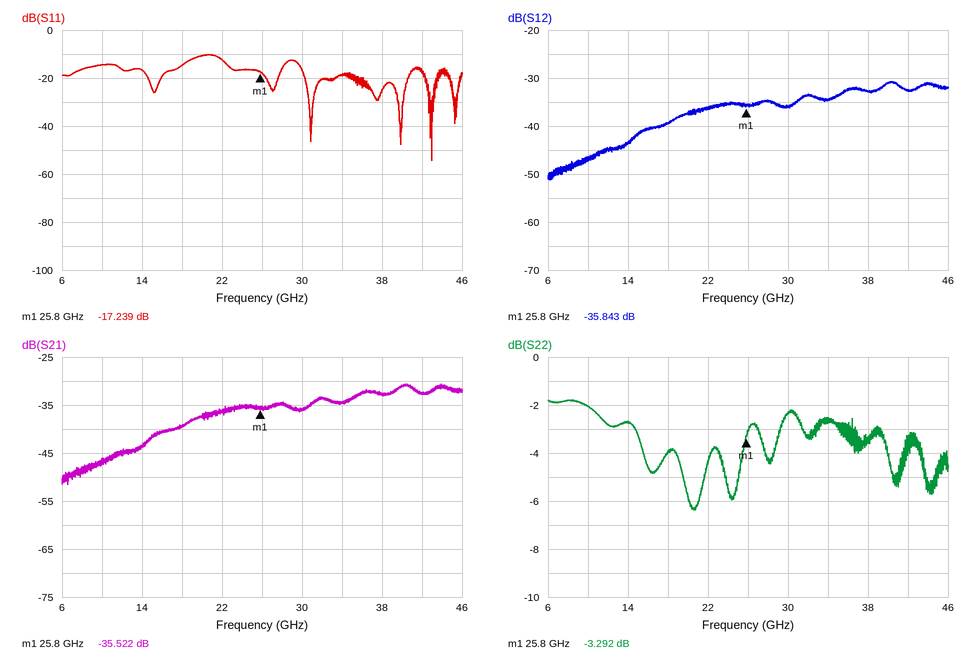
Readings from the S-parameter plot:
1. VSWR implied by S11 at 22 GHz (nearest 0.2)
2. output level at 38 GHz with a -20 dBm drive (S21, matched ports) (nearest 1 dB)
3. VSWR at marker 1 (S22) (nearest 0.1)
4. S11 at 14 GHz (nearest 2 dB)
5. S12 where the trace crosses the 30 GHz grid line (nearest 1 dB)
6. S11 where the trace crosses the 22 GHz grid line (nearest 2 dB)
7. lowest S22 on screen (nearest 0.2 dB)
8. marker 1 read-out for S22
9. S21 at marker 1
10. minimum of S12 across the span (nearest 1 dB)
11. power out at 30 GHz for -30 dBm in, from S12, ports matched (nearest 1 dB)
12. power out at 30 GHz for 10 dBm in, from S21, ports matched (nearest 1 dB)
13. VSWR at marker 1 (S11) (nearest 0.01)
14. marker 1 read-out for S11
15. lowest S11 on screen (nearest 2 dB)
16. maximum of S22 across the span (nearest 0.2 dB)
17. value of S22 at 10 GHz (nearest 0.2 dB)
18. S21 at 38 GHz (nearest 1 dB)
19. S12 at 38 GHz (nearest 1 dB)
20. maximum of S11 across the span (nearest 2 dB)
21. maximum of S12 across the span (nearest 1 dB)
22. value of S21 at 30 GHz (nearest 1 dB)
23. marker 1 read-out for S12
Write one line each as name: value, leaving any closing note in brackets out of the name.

VSWR implied by S11 at 22 GHz: 1.6
output level at 38 GHz with a -20 dBm drive (S21, matched ports): -53 dBm
VSWR at marker 1 (S22): 5.3
S11 at 14 GHz: -16 dB
S12 where the trace crosses the 30 GHz grid line: -36 dB
S11 where the trace crosses the 22 GHz grid line: -12 dB
lowest S22 on screen: -6.4 dB
marker 1 read-out for S22: -3.292 dB
S21 at marker 1: -35.522 dB
minimum of S12 across the span: -51 dB
power out at 30 GHz for -30 dBm in, from S12, ports matched: -66 dBm
power out at 30 GHz for 10 dBm in, from S21, ports matched: -26 dBm
VSWR at marker 1 (S11): 1.32
marker 1 read-out for S11: -17.239 dB
lowest S11 on screen: -54 dB
maximum of S22 across the span: -1.8 dB
value of S22 at 10 GHz: -2.0 dB
S21 at 38 GHz: -33 dB
S12 at 38 GHz: -33 dB
maximum of S11 across the span: -10 dB
maximum of S12 across the span: -31 dB
value of S21 at 30 GHz: -36 dB
marker 1 read-out for S12: -35.843 dB
